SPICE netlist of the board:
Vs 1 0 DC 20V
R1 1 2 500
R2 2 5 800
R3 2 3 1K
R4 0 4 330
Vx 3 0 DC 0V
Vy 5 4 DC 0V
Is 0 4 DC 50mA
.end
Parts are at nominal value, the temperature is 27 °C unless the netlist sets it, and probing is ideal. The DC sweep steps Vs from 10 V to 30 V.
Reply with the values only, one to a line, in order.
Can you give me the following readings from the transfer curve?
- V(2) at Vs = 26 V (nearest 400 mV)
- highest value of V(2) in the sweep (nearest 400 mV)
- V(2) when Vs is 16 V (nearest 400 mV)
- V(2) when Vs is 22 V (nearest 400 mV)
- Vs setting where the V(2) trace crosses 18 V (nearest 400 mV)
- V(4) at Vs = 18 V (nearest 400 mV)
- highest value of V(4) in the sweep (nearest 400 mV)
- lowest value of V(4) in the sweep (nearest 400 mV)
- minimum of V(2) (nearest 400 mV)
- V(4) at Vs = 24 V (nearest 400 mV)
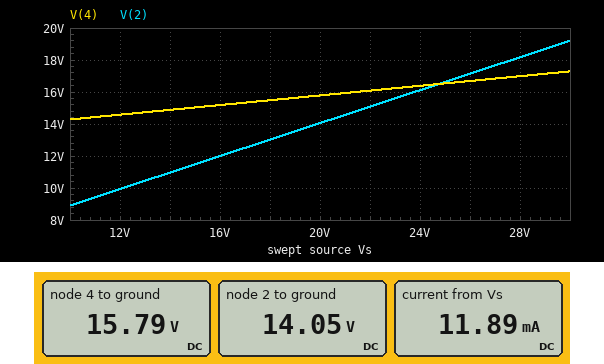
17.2 V
19.2 V
12.0 V
15.2 V
27.6 V
15.6 V
17.2 V
14.4 V
8.8 V
16.4 V
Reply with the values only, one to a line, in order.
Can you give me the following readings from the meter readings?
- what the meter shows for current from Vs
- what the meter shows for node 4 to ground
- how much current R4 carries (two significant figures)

11.89 mA
15.79 V
48 mA
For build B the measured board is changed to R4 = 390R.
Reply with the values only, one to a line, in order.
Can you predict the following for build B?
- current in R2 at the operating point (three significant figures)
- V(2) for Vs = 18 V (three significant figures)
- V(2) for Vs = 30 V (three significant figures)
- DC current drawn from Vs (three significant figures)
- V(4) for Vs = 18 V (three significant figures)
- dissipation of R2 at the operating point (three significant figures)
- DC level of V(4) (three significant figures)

4.05 mA
13.6 V
19.9 V
10.6 mA
17.6 V
13.1 mW
17.9 V
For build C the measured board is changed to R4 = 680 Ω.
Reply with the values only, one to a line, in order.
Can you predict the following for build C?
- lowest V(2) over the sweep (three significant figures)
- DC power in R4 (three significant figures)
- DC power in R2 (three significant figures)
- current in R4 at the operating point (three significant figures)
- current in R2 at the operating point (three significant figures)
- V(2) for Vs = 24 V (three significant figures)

11.7 V
1.01 W
104 mW
38.6 mA
11.4 mA
19.3 V
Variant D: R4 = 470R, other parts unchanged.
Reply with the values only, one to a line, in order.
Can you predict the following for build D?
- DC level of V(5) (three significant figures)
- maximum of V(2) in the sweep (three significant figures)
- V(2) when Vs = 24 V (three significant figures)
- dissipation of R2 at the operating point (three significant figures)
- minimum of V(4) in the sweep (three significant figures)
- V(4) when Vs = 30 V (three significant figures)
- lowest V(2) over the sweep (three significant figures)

20.5 V
20.7 V
17.6 V
32.2 mW
18.6 V
22.5 V
10.2 V
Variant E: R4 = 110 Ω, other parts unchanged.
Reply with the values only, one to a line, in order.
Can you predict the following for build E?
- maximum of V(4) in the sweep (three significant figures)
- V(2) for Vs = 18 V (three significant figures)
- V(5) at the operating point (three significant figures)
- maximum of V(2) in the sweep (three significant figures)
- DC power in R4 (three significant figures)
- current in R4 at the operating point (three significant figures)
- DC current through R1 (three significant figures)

6.78 V
10.3 V
6.19 V
16.1 V
349 mW
56.3 mA
17.5 mA
